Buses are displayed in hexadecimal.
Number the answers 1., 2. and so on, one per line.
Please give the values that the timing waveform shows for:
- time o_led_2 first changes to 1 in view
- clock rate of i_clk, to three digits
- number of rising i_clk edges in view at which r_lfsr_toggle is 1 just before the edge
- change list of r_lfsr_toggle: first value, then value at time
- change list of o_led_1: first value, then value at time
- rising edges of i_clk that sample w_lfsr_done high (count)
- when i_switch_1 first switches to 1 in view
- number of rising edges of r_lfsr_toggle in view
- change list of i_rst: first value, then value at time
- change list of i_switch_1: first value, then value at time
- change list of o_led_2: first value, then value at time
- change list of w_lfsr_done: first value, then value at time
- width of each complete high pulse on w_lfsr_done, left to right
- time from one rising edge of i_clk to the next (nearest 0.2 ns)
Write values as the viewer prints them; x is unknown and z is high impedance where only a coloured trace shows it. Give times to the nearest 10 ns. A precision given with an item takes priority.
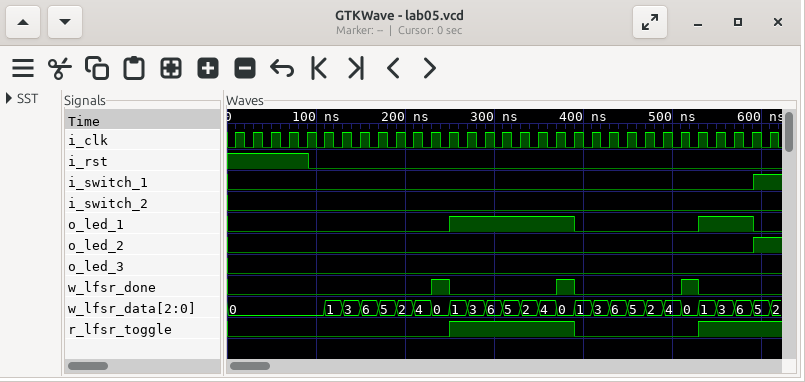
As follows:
1. 590 ns
2. 50.0 MHz
3. 11
4. 0, 1 at 250 ns, 0 at 390 ns, 1 at 530 ns
5. 0, 1 at 250 ns, 0 at 390 ns, 1 at 530 ns, 0 at 590 ns
6. 3
7. 590 ns
8. 2
9. 1, 0 at 90 ns
10. 0, 1 at 590 ns
11. 0, 1 at 590 ns
12. 0, 1 at 230 ns, 0 at 250 ns, 1 at 370 ns, 0 at 390 ns, 1 at 510 ns, 0 at 530 ns
13. 20 ns, 20 ns, 20 ns
14. 20 ns
